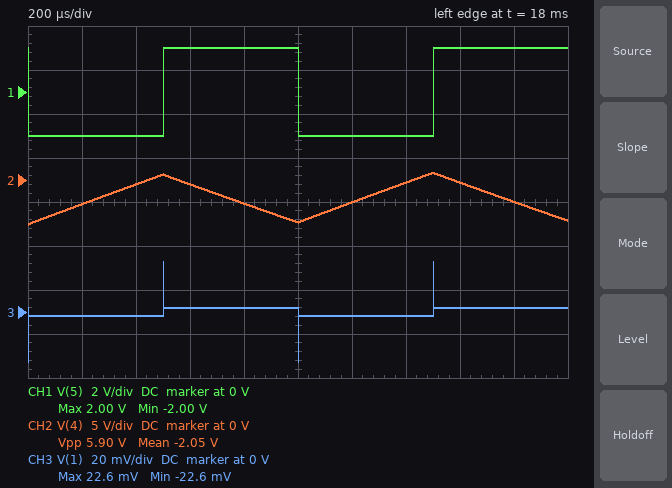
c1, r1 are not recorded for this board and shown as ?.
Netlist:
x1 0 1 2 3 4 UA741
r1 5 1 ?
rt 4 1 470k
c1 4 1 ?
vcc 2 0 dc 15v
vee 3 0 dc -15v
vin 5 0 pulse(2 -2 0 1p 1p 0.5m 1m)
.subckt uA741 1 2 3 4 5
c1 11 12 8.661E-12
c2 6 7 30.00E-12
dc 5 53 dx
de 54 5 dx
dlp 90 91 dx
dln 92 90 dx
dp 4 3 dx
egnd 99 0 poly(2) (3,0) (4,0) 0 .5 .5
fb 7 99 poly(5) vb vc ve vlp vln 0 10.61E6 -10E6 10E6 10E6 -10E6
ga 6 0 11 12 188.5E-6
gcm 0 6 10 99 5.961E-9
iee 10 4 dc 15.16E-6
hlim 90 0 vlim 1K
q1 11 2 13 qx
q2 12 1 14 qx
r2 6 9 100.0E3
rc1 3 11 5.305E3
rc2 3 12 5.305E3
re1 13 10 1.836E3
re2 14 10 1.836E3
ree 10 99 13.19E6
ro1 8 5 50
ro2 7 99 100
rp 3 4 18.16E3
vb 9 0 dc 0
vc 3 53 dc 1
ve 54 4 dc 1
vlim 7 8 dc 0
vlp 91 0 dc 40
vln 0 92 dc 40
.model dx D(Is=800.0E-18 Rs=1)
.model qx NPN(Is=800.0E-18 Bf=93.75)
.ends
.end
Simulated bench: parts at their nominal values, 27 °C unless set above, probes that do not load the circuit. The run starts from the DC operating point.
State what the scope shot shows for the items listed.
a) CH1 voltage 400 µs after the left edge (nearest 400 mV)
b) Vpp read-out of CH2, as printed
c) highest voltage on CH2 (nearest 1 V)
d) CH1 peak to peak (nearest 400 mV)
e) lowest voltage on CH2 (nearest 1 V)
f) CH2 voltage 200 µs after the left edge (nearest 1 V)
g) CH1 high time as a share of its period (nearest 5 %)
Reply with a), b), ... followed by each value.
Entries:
a) -2.0 V
b) 5.90 V
c) 1 V
d) 4.0 V
e) -5 V
f) -3 V
g) 50 %
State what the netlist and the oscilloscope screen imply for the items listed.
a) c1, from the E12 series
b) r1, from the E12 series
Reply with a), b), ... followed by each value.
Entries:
a) 22 nF
b) 8.2 kΩ
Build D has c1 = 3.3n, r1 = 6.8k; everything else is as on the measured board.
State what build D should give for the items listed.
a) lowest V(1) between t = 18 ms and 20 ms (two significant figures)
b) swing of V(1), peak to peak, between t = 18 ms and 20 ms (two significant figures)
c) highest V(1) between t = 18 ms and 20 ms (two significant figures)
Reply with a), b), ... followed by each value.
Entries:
a) -1.8 V
b) 3.5 V
c) 1.8 V
